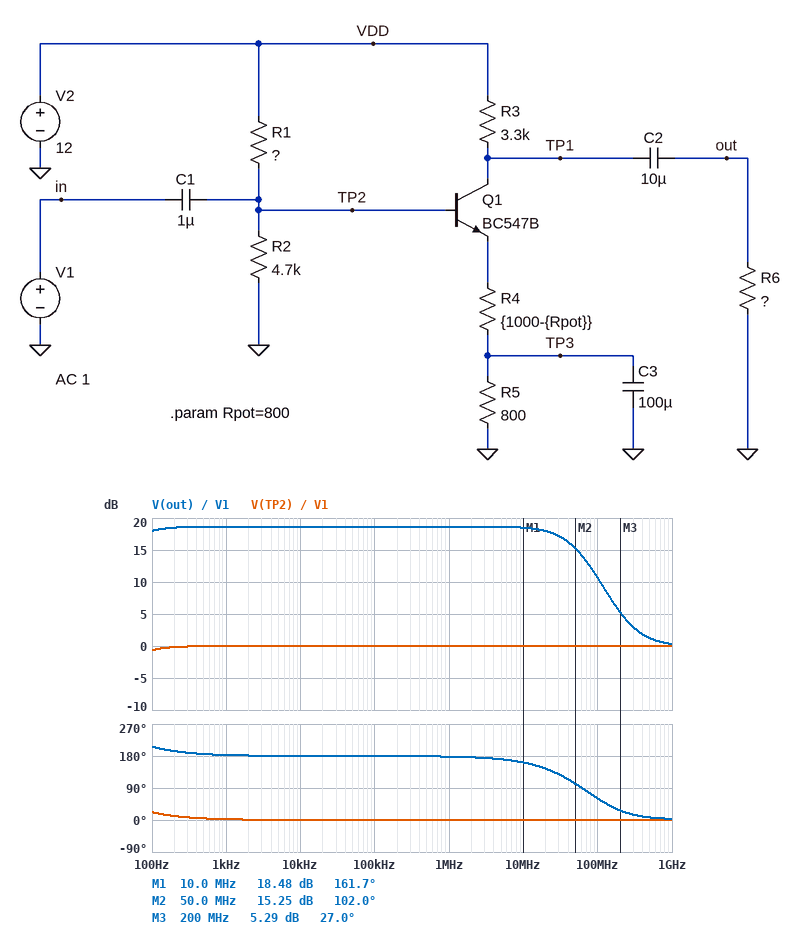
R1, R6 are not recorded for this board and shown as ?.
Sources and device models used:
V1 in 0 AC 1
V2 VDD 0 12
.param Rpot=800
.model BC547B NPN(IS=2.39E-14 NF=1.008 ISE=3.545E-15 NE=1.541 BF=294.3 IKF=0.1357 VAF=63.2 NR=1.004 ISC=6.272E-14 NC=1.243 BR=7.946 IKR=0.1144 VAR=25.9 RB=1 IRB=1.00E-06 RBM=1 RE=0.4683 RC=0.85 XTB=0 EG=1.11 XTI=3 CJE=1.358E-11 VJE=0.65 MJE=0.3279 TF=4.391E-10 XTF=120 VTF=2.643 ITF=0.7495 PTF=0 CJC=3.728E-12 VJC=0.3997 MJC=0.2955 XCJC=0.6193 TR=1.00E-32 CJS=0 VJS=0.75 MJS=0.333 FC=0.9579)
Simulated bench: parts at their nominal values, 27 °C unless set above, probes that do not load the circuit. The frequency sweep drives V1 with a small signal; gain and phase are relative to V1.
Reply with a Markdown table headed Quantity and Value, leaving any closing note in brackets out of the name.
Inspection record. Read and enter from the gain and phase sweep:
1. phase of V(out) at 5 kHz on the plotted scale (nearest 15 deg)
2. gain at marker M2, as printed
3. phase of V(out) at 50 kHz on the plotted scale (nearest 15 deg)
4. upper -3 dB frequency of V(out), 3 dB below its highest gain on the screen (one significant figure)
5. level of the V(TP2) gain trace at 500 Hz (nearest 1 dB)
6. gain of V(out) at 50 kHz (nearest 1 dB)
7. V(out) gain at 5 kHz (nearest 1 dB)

| Quantity | Value |
|---|---|
| phase of V(out) at 5 kHz on the plotted scale | 180 deg |
| gain at marker M2, as printed | 15.25 dB |
| phase of V(out) at 50 kHz on the plotted scale | 180 deg |
| upper -3 dB frequency of V(out), 3 dB below its highest gain on the screen | 50 MHz |
| level of the V(TP2) gain trace at 500 Hz | 0 dB |
| gain of V(out) at 50 kHz | 19 dB |
| V(out) gain at 5 kHz | 19 dB |
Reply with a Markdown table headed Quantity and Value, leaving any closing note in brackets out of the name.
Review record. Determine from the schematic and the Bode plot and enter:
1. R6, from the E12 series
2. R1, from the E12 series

| Quantity | Value |
|---|---|
| R6, from the E12 series | 5.6 kΩ |
| R1, from the E12 series | 39 kΩ |
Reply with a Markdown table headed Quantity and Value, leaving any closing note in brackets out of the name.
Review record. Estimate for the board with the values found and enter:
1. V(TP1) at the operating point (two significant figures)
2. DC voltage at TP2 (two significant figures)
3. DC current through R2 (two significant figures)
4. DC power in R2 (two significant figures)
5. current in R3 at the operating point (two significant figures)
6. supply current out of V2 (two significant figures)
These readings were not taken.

| Quantity | Value |
|---|---|
| V(TP1) at the operating point | 9.8 V |
| DC voltage at TP2 | 1.3 V |
| DC current through R2 | 270 µA |
| DC power in R2 | 350 µW |
| current in R3 at the operating point | 660 µA |
| supply current out of V2 | 930 µA |
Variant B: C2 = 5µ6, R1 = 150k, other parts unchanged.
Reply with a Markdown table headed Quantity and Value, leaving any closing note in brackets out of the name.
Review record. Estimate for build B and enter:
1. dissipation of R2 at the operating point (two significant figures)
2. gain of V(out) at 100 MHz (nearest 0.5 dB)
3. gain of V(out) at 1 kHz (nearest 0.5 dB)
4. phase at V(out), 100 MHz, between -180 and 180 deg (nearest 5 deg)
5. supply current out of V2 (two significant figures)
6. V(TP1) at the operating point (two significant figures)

| Quantity | Value |
|---|---|
| dissipation of R2 at the operating point | 28 µW |
| gain of V(out) at 100 MHz | -1.0 dB |
| gain of V(out) at 1 kHz | -51.5 dB |
| phase at V(out), 100 MHz, between -180 and 180 deg | 30 deg |
| supply current out of V2 | 78 µA |
| V(TP1) at the operating point | 12 V |
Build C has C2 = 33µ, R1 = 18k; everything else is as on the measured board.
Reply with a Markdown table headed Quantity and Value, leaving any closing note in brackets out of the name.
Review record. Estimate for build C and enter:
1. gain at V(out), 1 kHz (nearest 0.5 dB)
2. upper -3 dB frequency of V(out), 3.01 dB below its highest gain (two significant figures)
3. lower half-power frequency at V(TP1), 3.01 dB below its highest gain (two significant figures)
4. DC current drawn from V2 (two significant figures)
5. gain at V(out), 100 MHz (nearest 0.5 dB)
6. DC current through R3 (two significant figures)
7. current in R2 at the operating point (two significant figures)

| Quantity | Value |
|---|---|
| gain at V(out), 1 kHz | 19.5 dB |
| upper -3 dB frequency of V(out), 3.01 dB below its highest gain | 40 MHz |
| lower half-power frequency at V(TP1), 3.01 dB below its highest gain | 47 Hz |
| DC current drawn from V2 | 2.3 mA |
| gain at V(out), 100 MHz | 11.0 dB |
| DC current through R3 | 1.8 mA |
| current in R2 at the operating point | 520 µA |
